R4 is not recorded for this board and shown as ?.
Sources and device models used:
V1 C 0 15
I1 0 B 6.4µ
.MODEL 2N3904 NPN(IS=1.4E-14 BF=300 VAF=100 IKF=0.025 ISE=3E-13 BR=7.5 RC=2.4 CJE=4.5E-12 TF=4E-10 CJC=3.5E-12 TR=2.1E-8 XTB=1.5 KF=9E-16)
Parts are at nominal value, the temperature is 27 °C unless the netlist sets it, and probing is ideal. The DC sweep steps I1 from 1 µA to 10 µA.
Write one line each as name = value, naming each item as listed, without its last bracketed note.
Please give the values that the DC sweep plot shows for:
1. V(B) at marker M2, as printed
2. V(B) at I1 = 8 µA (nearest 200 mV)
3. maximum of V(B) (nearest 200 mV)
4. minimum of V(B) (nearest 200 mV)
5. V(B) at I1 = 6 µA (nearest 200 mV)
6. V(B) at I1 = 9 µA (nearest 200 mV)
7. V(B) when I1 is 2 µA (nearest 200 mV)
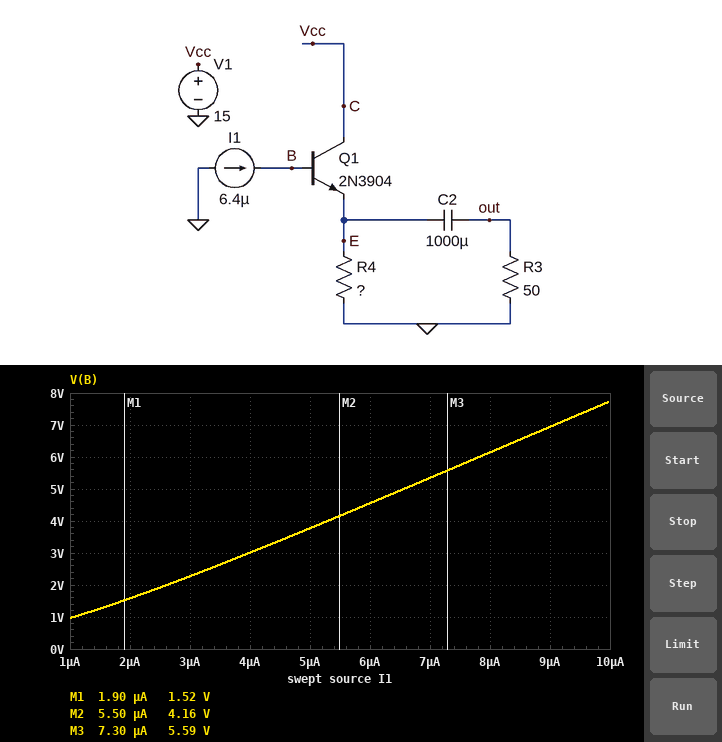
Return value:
V(B) at marker M2, as printed = 4.16 V
V(B) at I1 = 8 µA = 6.2 V
maximum of V(B) = 7.8 V
minimum of V(B) = 1.0 V
V(B) at I1 = 6 µA = 4.6 V
V(B) at I1 = 9 µA = 7.0 V
V(B) when I1 is 2 µA = 1.6 V
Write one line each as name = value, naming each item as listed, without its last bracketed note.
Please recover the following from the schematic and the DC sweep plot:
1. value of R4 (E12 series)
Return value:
value of R4 = 5.6 kΩ
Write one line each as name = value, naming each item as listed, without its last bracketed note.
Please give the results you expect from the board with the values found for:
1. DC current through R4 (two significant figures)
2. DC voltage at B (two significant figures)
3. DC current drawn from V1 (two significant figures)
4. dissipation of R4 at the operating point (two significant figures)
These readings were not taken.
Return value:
DC current through R4 = 760 µA
DC voltage at B = 4.9 V
DC current drawn from V1 = 750 µA
dissipation of R4 at the operating point = 3.2 mW
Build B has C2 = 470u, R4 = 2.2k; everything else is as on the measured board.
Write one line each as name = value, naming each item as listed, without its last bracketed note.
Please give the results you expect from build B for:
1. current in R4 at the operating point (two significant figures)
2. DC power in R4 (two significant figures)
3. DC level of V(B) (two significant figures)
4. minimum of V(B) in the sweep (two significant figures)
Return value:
current in R4 at the operating point = 770 µA
DC power in R4 = 1.3 mW
DC level of V(B) = 2.3 V
minimum of V(B) in the sweep = 730 mV
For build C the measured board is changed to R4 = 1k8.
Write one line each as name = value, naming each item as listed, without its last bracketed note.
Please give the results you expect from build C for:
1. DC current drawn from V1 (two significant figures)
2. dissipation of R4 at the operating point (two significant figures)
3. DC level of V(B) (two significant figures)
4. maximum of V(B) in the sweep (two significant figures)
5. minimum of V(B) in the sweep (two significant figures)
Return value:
DC current drawn from V1 = 770 µA
dissipation of R4 at the operating point = 1.1 mW
DC level of V(B) = 2.0 V
maximum of V(B) in the sweep = 3.0 V
minimum of V(B) in the sweep = 700 mV
